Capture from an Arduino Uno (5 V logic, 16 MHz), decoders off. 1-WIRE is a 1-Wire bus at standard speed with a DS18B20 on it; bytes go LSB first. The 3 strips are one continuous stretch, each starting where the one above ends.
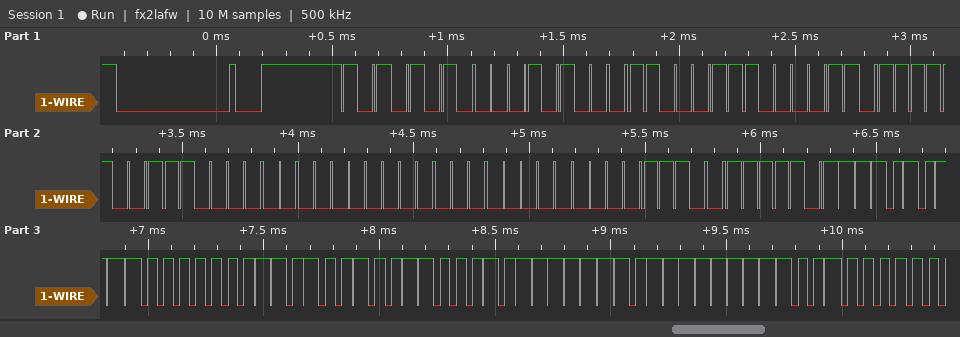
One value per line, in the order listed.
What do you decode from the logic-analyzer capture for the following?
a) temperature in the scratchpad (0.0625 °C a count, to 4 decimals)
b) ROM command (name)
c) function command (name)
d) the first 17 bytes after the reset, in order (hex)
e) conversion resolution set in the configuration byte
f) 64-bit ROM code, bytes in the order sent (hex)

29.4375 °C
Match ROM
Read Scratchpad
55 28 C6 61 9F 03 00 00 70 BE D7 01 4B 46 7F FF 09
12 bits
28 C6 61 9F 03 00 00 70
